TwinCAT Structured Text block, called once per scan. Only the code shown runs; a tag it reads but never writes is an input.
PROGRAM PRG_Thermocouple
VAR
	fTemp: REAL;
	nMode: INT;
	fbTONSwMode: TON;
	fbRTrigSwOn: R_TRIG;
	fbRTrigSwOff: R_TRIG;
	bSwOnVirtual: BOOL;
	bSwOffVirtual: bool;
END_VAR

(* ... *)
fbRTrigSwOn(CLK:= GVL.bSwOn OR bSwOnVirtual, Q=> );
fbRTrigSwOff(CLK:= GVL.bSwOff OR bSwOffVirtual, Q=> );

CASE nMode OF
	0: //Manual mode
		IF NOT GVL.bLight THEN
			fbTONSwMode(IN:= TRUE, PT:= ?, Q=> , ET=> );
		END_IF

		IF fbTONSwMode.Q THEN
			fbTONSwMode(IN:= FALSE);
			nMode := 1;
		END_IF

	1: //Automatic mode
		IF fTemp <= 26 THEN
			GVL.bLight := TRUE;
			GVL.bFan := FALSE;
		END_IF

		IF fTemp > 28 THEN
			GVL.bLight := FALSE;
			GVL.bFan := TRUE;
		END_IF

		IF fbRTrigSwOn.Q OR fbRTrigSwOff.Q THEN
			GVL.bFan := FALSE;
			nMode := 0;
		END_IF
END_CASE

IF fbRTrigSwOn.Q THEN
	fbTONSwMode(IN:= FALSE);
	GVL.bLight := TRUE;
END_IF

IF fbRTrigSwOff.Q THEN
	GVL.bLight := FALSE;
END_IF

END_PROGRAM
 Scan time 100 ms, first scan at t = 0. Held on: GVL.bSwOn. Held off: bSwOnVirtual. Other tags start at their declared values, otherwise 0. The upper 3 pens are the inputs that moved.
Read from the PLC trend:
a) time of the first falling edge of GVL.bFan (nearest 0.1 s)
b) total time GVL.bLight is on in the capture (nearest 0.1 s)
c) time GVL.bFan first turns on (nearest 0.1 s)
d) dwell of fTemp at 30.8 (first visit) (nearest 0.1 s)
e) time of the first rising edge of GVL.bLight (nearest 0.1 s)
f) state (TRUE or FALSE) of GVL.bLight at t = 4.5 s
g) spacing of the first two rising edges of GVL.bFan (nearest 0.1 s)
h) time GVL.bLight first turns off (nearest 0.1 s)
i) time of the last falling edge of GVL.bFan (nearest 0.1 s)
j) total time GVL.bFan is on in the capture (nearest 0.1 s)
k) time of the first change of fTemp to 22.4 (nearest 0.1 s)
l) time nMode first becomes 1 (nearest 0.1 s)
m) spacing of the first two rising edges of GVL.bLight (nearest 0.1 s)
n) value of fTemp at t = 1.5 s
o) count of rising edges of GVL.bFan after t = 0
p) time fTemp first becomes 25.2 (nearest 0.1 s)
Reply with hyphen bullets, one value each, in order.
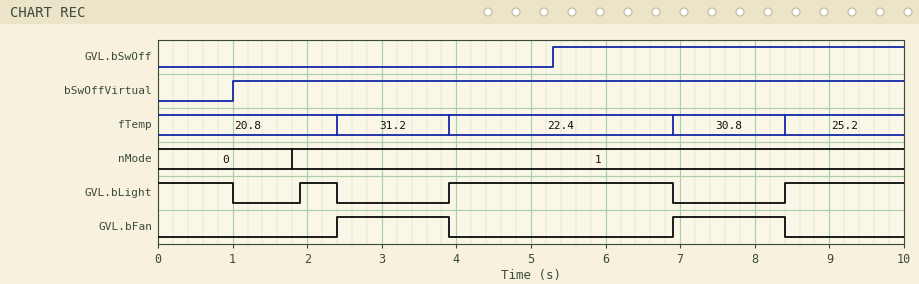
- 3.9 s
- 6.1 s
- 2.4 s
- 1.5 s
- 1.9 s
- TRUE
- 4.5 s
- 1.0 s
- 8.4 s
- 3.0 s
- 3.9 s
- 1.8 s
- 2.0 s
- 20.8
- 2
- 8.4 s
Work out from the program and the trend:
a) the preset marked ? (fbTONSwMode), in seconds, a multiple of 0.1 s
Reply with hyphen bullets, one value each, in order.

- 0.7 s
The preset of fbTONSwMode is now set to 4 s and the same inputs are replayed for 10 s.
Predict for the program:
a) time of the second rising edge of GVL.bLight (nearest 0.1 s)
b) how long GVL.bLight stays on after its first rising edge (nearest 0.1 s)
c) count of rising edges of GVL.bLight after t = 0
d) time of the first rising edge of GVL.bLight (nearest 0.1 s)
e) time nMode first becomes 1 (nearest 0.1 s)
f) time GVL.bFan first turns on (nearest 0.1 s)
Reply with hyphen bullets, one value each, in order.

- 8.4 s
- 1.7 s
- 2
- 5.2 s
- 5.1 s
- 6.9 s
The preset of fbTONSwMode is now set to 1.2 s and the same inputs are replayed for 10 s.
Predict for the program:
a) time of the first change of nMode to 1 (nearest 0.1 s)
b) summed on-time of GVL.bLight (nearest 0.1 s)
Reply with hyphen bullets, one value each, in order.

- 2.3 s
- 5.6 s
